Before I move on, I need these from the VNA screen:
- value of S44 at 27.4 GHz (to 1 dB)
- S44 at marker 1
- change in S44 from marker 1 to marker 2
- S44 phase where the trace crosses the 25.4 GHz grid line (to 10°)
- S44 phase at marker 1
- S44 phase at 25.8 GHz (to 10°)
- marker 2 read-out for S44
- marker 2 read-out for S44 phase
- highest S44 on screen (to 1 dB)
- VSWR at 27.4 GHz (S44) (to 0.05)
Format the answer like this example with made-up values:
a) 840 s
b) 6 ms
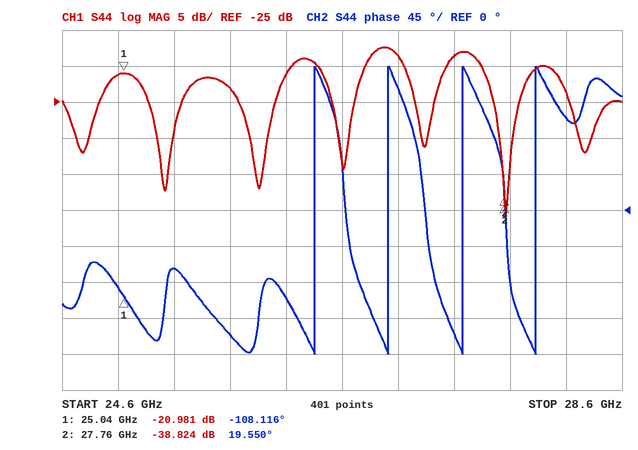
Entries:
a) -19 dB
b) -20.981 dB
c) -17.843 dB
d) -70°
e) -108.116°
f) -160°
g) -38.824 dB
h) 19.550°
i) -17 dB
j) 1.25
